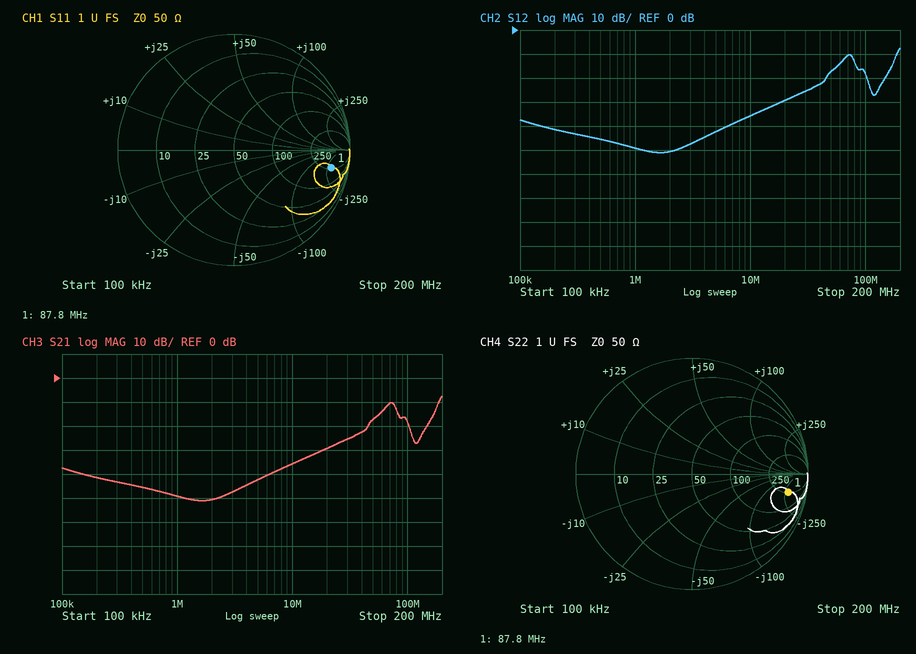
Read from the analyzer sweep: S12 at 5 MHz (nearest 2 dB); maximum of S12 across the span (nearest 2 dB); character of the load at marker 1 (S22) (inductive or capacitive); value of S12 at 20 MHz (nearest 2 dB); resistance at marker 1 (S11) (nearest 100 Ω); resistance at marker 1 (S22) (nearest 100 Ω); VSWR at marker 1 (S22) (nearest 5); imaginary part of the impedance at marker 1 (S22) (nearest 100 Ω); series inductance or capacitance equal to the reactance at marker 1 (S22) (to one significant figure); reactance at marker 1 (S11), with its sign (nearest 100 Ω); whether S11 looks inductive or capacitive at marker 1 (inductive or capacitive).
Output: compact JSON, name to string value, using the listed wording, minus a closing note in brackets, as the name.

{"S12 at 5 MHz": "-42 dB", "maximum of S12 across the span": "-8 dB", "character of the load at marker 1 (S22)": "capacitive", "value of S12 at 20 MHz": "-30 dB", "resistance at marker 1 (S11)": "300 Ω", "resistance at marker 1 (S22)": "300 Ω", "VSWR at marker 1 (S22)": "10", "imaginary part of the impedance at marker 1 (S22)": "-300 Ω", "series inductance or capacitance equal to the reactance at marker 1 (S22)": "6 pF", "reactance at marker 1 (S11), with its sign": "-300 Ω", "whether S11 looks inductive or capacitive at marker 1": "capacitive"}
